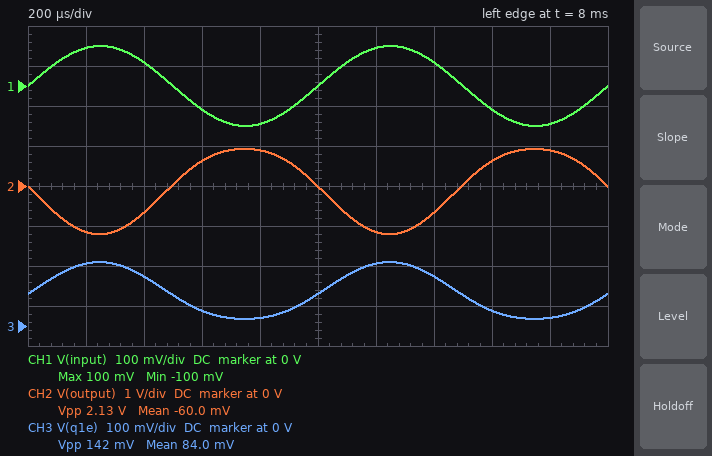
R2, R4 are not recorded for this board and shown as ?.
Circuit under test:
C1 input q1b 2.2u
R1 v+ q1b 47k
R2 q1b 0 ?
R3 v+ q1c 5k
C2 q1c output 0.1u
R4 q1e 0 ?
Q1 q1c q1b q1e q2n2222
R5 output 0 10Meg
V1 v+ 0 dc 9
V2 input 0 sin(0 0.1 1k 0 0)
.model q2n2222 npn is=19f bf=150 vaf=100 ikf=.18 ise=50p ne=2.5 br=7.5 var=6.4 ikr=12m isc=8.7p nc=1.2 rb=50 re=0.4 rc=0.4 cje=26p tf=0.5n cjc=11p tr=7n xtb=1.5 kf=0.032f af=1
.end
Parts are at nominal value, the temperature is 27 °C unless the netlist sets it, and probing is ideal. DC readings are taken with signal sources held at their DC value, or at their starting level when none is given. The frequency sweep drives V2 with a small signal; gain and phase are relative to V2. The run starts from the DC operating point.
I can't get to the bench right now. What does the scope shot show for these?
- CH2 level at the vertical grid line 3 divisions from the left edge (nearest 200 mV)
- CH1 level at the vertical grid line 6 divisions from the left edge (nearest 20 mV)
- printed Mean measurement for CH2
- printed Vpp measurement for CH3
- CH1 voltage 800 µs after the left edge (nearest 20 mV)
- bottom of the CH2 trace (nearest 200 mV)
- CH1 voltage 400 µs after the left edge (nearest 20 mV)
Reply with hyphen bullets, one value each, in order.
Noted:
- 600 mV
- 100 mV
- -60.0 mV
- 142 mV
- -100 mV
- -1.2 V
- 60 mV
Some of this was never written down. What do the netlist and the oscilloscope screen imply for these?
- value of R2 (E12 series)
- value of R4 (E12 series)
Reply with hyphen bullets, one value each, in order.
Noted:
- 3.9 kΩ
- 330 Ω
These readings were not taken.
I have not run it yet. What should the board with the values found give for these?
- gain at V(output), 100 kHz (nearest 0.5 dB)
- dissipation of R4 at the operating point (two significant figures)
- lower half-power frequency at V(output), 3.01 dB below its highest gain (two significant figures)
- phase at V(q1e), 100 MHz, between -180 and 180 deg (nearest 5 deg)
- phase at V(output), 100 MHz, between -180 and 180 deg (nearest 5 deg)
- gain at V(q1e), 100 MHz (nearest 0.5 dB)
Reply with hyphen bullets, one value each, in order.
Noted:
- 21.0 dB
- 19 µW
- 21 Hz
- 5 deg
- 10 deg
- -1.5 dB
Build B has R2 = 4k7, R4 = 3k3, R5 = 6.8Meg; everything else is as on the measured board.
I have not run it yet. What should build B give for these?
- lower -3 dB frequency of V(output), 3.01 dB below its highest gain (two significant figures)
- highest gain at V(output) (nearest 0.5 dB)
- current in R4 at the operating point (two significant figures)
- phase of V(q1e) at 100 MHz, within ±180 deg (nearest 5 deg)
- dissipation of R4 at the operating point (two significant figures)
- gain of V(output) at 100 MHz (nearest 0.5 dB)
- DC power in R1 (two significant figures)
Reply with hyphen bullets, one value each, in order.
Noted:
- 17 Hz
- 2.5 dB
- 74 µA
- 0 deg
- 18 µW
- 0 dB
- 1.4 mW
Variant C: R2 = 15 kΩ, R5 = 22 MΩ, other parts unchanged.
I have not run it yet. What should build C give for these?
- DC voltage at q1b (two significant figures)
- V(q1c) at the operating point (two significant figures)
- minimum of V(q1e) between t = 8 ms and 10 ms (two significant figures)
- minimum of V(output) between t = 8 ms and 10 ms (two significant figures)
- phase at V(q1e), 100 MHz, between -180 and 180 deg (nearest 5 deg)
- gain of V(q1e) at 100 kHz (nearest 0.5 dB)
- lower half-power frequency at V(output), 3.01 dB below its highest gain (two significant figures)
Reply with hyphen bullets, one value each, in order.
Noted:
- 1.2 V
- 740 mV
- 450 mV
- -2.8 mV
- 0 deg
- -1.5 dB
- 19 MHz
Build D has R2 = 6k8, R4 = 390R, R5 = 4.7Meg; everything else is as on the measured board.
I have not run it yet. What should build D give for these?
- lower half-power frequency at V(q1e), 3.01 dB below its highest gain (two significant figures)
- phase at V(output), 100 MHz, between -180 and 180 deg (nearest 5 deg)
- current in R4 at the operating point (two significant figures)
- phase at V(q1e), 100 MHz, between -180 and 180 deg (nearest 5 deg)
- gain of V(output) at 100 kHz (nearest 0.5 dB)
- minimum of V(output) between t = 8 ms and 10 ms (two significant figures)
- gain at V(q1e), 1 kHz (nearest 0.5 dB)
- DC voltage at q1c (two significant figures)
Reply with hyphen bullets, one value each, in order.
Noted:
- 14 Hz
- 15 deg
- 1.1 mA
- 0 deg
- 21.5 dB
- -1.2 V
- -0.5 dB
- 3.4 V
